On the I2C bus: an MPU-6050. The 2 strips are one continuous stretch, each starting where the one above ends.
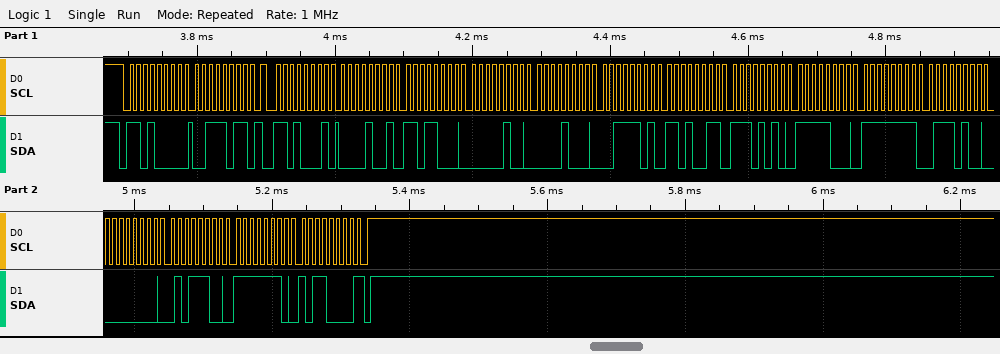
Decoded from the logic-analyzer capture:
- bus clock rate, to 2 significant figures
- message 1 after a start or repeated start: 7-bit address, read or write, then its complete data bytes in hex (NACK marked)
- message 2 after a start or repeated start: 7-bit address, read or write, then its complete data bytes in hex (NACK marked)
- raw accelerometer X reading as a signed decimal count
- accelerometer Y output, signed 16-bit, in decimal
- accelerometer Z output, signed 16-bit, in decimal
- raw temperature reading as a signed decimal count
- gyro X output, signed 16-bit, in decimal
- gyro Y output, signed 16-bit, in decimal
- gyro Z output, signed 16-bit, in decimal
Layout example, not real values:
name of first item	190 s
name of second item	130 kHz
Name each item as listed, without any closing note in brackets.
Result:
bus clock rate, to 2 significant figures	100 kHz
message 1 after a start or repeated start: 7-bit address, read or write, then its complete data bytes in hex	0x68 write: 3B
message 2 after a start or repeated start: 7-bit address, read or write, then its complete data bytes in hex	0x68 read: 09 D8 04 08 3D D3 EA F8 FF 74 00 5C FE B0 NACK
raw accelerometer X reading as a signed decimal count	2520
accelerometer Y output, signed 16-bit, in decimal	1032
accelerometer Z output, signed 16-bit, in decimal	15827
raw temperature reading as a signed decimal count	-5384
gyro X output, signed 16-bit, in decimal	-140
gyro Y output, signed 16-bit, in decimal	92
gyro Z output, signed 16-bit, in decimal	-336
